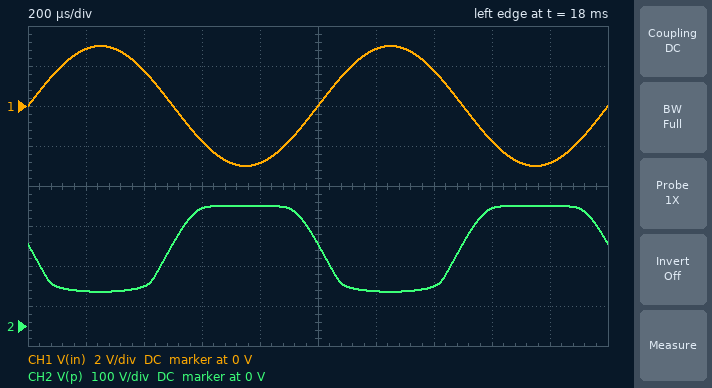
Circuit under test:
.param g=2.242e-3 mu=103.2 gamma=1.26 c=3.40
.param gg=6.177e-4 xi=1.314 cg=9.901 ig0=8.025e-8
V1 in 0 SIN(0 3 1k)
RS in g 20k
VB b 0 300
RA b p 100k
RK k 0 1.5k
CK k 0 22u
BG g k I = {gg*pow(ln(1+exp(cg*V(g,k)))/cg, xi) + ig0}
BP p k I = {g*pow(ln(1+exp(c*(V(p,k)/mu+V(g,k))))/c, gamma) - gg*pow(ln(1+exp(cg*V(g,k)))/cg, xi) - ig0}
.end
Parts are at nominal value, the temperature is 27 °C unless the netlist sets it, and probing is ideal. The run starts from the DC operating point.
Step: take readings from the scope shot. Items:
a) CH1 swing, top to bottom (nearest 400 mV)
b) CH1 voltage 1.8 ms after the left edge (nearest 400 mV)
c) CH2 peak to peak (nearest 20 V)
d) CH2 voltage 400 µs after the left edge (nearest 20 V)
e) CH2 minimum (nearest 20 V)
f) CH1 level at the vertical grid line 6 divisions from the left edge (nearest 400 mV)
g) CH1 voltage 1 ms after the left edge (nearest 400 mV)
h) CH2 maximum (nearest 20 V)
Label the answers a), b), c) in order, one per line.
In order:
a) 6.0 V
b) -2.8 V
c) 220 V
d) 100 V
e) 80 V
f) 2.8 V
g) 0 V
h) 300 V
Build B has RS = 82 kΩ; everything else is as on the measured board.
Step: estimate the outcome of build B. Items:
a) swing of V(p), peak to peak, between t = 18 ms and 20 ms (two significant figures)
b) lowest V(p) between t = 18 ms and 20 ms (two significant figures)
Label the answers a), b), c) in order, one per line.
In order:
a) 200 V
b) 97 V
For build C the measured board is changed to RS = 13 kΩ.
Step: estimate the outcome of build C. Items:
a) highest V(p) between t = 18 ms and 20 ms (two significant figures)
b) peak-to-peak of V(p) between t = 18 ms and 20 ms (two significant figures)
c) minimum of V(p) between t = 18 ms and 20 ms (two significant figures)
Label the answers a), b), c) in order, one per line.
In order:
a) 300 V
b) 220 V
c) 81 V
